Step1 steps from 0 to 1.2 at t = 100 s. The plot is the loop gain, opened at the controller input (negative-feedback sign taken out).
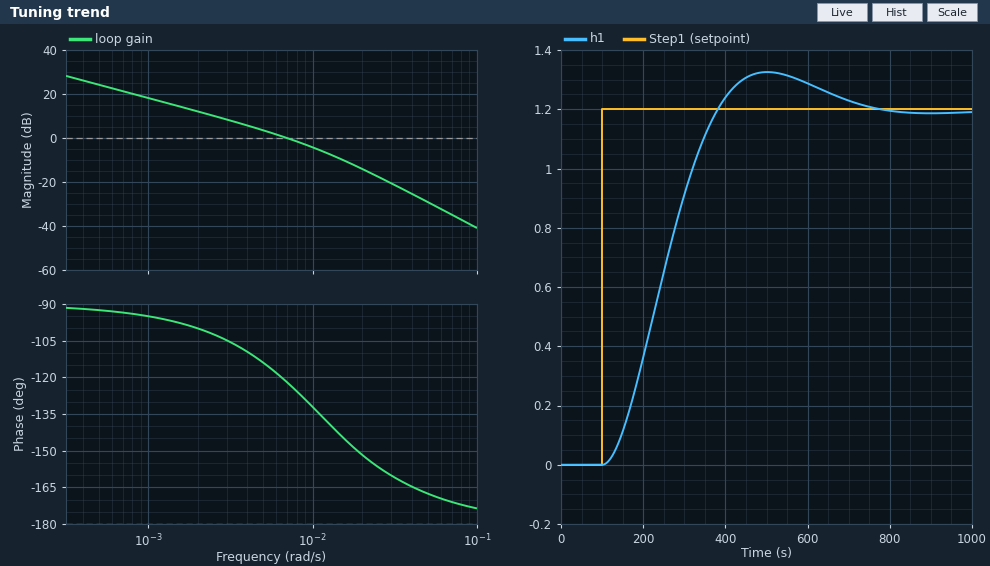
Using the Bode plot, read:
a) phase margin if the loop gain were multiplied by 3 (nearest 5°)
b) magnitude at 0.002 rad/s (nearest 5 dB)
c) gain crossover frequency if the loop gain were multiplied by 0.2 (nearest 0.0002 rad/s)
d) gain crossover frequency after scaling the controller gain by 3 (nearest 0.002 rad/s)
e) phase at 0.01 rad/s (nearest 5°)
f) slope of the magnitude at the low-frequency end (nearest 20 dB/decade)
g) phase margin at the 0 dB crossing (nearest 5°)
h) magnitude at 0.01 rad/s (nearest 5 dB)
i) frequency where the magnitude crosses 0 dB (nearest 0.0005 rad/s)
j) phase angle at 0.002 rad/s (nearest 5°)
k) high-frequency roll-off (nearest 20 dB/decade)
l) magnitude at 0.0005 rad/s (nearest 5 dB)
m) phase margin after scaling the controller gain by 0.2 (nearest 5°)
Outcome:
35°
10 dB
0.0016 rad/s
0.014 rad/s
-130°
-20 dB/decade
60°
-5 dB
0.0070 rad/s
-100°
-40 dB/decade
25 dB
80°
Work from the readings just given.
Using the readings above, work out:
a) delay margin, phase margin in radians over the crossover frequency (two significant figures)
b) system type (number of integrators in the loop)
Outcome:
150 s
1
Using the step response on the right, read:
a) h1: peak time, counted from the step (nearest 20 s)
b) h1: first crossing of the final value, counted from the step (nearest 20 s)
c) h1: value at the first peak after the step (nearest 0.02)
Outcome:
400 s
280 s
1.32
